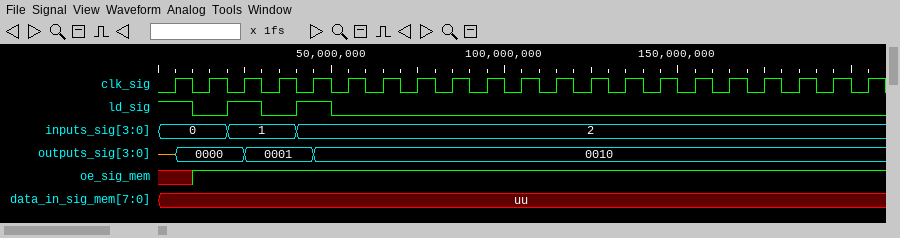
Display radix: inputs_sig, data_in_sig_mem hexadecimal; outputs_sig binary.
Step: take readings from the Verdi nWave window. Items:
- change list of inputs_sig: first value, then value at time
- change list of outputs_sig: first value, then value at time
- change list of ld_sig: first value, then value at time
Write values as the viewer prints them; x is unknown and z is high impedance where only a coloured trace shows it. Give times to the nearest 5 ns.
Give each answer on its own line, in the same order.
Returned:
0, 1 at 20 ns, 2 at 40 ns
z, 0000 at 5 ns, 0001 at 25 ns, 0010 at 45 ns
1, 0 at 10 ns, 1 at 20 ns, 0 at 30 ns, 1 at 40 ns, 0 at 50 ns
